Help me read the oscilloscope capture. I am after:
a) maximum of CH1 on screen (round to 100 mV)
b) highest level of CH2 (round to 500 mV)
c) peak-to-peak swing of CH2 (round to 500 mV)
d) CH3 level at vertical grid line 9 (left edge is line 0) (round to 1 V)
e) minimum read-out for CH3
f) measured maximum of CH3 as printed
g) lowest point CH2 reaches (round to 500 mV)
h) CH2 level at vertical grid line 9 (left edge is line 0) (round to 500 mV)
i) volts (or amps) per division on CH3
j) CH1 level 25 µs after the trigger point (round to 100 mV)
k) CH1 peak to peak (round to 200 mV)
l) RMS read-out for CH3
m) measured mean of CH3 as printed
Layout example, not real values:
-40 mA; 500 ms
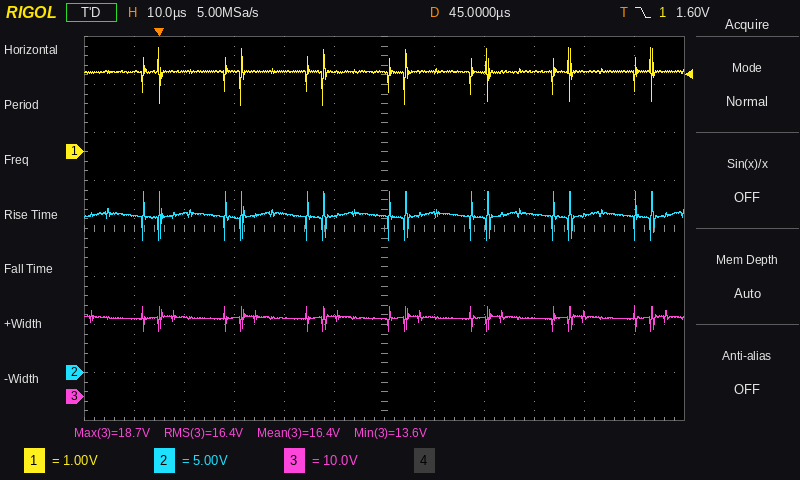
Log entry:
2.2 V; 19.0 V; 5.0 V; 16 V; 13.6 V; 18.7 V; 14.0 V; 16.5 V; 10 V; 1.7 V; 1.2 V; 16.4 V; 16.4 V
